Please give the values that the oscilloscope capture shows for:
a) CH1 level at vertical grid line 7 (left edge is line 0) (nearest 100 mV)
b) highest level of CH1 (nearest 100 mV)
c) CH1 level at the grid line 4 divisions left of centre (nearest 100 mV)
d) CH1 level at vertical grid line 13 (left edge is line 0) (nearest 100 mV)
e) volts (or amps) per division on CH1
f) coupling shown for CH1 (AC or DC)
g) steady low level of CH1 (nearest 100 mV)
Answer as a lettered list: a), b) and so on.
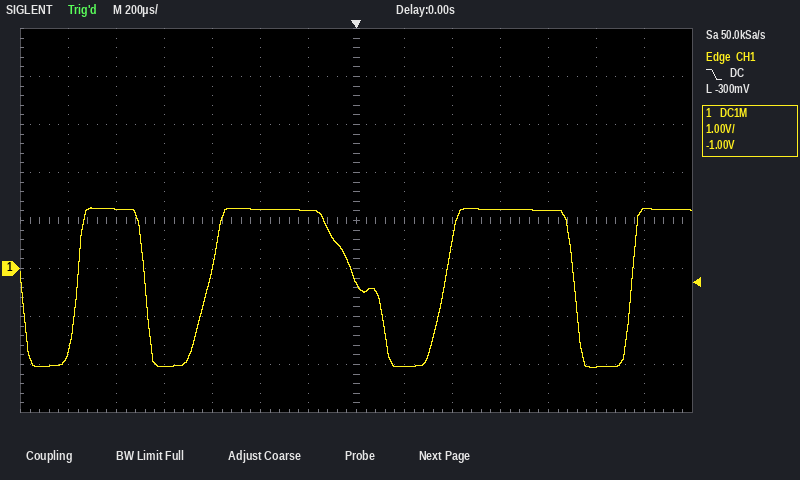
a) -300 mV
b) 1.3 V
c) -2.0 V
d) 1.2 V
e) 1 V
f) DC
g) -2.0 V
